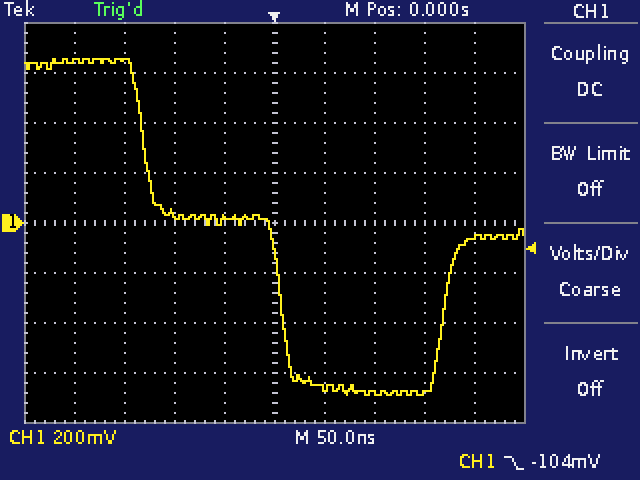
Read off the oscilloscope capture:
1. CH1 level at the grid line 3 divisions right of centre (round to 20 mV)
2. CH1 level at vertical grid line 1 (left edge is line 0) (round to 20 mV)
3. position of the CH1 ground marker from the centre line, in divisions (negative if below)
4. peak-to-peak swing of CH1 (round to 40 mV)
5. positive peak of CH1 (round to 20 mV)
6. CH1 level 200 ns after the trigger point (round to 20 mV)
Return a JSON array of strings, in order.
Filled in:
["-680 mV", "640 mV", "0.0 div", "1.36 V", "660 mV", "-60 mV"]
